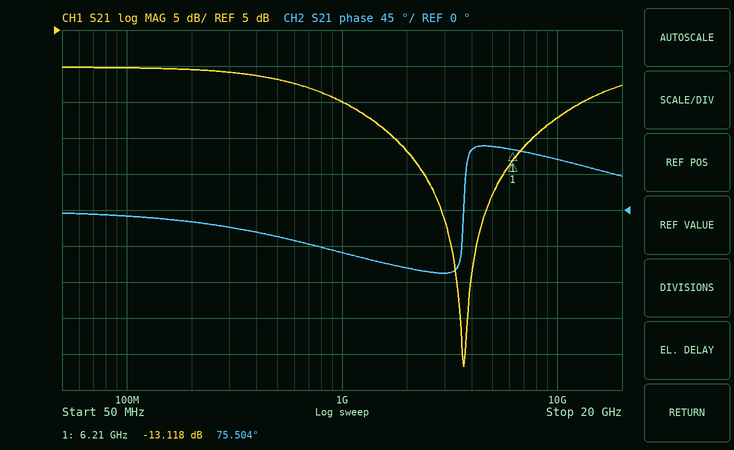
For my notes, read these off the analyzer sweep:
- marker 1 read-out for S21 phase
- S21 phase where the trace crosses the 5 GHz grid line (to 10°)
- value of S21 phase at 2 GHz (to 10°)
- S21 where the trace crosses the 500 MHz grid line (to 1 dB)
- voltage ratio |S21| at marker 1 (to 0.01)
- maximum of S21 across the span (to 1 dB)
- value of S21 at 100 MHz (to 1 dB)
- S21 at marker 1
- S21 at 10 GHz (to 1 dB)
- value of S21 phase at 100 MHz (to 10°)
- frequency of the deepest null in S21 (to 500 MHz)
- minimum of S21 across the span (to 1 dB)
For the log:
75.504°
80°
-70°
-2 dB
0.22
0 dB
0 dB
-13.118 dB
-7 dB
-10°
3.5 GHz
-42 dB
